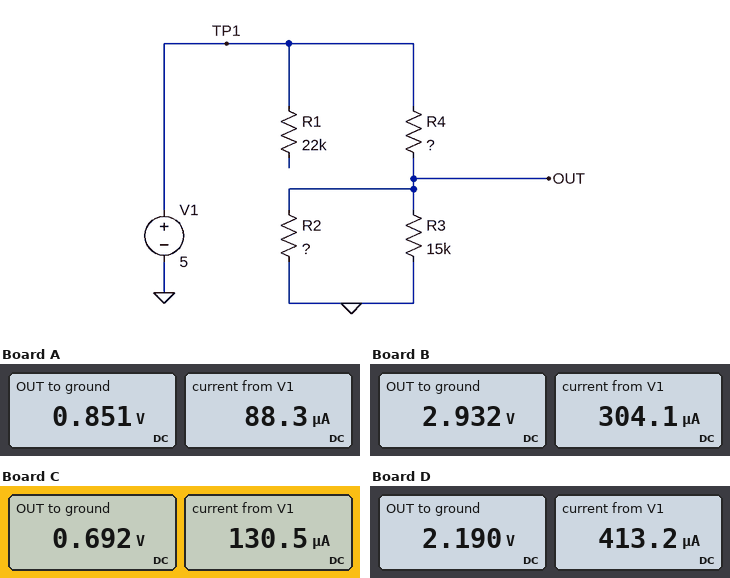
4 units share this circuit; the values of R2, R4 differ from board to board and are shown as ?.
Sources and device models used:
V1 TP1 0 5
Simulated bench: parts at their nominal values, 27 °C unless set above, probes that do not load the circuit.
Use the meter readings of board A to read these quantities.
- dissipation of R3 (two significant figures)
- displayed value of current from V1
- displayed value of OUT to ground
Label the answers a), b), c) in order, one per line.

a) 48 µW
b) 88.3 µA
c) 0.851 V
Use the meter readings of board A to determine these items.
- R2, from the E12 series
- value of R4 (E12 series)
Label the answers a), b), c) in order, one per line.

a) 27 kΩ
b) 47 kΩ
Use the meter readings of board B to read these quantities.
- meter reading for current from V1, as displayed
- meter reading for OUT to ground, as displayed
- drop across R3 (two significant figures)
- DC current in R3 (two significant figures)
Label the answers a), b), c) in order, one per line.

a) 304.1 µA
b) 2.932 V
c) 2.9 V
d) 200 µA
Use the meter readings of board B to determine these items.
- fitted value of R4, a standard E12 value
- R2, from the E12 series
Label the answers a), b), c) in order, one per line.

a) 6.8 kΩ
b) 27 kΩ
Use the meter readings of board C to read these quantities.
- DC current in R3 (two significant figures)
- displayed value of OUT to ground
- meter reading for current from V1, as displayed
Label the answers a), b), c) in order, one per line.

a) 46 µA
b) 0.692 V
c) 130.5 µA
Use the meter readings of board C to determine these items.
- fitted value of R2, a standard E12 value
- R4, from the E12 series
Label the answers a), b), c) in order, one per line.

a) 8.2 kΩ
b) 33 kΩ
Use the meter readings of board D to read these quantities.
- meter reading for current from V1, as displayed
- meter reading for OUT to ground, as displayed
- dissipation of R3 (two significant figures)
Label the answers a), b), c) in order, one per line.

a) 413.2 µA
b) 2.190 V
c) 320 µW
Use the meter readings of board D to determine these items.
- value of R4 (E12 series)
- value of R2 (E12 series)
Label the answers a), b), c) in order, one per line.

a) 6.8 kΩ
b) 8.2 kΩ
